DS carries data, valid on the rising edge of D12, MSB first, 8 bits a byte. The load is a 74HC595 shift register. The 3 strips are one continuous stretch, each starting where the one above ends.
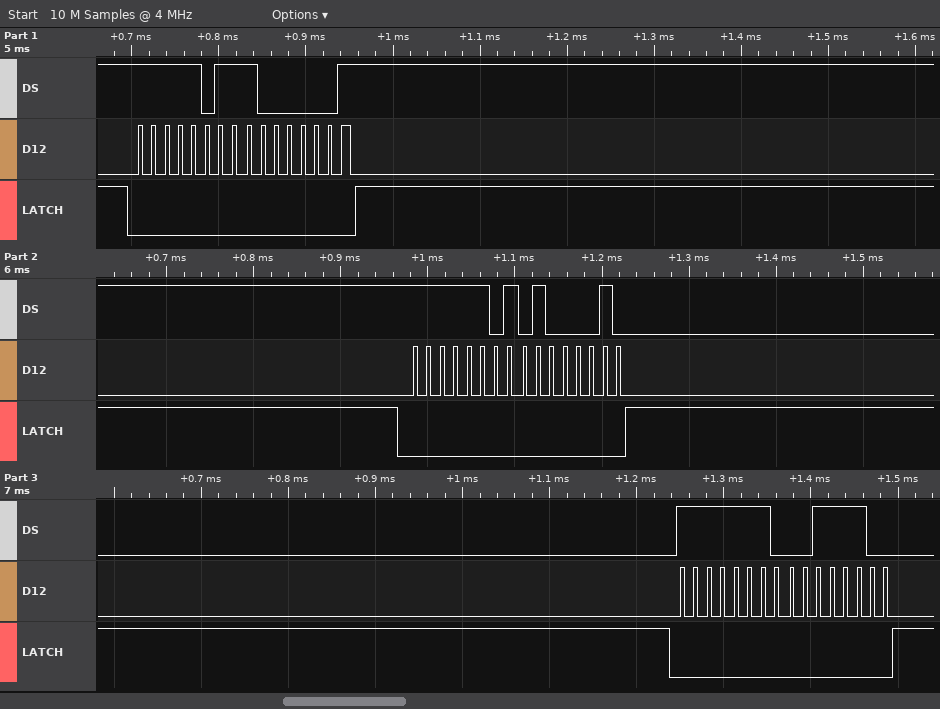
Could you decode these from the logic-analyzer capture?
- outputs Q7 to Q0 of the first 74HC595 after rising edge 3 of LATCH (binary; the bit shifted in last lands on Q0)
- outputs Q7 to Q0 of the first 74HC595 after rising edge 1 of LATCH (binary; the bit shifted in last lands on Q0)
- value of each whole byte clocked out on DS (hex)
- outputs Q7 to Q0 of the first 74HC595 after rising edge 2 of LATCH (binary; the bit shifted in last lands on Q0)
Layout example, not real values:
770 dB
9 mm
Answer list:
00111100
10000001
FB 81 FD 42 FE 3C
01000010
